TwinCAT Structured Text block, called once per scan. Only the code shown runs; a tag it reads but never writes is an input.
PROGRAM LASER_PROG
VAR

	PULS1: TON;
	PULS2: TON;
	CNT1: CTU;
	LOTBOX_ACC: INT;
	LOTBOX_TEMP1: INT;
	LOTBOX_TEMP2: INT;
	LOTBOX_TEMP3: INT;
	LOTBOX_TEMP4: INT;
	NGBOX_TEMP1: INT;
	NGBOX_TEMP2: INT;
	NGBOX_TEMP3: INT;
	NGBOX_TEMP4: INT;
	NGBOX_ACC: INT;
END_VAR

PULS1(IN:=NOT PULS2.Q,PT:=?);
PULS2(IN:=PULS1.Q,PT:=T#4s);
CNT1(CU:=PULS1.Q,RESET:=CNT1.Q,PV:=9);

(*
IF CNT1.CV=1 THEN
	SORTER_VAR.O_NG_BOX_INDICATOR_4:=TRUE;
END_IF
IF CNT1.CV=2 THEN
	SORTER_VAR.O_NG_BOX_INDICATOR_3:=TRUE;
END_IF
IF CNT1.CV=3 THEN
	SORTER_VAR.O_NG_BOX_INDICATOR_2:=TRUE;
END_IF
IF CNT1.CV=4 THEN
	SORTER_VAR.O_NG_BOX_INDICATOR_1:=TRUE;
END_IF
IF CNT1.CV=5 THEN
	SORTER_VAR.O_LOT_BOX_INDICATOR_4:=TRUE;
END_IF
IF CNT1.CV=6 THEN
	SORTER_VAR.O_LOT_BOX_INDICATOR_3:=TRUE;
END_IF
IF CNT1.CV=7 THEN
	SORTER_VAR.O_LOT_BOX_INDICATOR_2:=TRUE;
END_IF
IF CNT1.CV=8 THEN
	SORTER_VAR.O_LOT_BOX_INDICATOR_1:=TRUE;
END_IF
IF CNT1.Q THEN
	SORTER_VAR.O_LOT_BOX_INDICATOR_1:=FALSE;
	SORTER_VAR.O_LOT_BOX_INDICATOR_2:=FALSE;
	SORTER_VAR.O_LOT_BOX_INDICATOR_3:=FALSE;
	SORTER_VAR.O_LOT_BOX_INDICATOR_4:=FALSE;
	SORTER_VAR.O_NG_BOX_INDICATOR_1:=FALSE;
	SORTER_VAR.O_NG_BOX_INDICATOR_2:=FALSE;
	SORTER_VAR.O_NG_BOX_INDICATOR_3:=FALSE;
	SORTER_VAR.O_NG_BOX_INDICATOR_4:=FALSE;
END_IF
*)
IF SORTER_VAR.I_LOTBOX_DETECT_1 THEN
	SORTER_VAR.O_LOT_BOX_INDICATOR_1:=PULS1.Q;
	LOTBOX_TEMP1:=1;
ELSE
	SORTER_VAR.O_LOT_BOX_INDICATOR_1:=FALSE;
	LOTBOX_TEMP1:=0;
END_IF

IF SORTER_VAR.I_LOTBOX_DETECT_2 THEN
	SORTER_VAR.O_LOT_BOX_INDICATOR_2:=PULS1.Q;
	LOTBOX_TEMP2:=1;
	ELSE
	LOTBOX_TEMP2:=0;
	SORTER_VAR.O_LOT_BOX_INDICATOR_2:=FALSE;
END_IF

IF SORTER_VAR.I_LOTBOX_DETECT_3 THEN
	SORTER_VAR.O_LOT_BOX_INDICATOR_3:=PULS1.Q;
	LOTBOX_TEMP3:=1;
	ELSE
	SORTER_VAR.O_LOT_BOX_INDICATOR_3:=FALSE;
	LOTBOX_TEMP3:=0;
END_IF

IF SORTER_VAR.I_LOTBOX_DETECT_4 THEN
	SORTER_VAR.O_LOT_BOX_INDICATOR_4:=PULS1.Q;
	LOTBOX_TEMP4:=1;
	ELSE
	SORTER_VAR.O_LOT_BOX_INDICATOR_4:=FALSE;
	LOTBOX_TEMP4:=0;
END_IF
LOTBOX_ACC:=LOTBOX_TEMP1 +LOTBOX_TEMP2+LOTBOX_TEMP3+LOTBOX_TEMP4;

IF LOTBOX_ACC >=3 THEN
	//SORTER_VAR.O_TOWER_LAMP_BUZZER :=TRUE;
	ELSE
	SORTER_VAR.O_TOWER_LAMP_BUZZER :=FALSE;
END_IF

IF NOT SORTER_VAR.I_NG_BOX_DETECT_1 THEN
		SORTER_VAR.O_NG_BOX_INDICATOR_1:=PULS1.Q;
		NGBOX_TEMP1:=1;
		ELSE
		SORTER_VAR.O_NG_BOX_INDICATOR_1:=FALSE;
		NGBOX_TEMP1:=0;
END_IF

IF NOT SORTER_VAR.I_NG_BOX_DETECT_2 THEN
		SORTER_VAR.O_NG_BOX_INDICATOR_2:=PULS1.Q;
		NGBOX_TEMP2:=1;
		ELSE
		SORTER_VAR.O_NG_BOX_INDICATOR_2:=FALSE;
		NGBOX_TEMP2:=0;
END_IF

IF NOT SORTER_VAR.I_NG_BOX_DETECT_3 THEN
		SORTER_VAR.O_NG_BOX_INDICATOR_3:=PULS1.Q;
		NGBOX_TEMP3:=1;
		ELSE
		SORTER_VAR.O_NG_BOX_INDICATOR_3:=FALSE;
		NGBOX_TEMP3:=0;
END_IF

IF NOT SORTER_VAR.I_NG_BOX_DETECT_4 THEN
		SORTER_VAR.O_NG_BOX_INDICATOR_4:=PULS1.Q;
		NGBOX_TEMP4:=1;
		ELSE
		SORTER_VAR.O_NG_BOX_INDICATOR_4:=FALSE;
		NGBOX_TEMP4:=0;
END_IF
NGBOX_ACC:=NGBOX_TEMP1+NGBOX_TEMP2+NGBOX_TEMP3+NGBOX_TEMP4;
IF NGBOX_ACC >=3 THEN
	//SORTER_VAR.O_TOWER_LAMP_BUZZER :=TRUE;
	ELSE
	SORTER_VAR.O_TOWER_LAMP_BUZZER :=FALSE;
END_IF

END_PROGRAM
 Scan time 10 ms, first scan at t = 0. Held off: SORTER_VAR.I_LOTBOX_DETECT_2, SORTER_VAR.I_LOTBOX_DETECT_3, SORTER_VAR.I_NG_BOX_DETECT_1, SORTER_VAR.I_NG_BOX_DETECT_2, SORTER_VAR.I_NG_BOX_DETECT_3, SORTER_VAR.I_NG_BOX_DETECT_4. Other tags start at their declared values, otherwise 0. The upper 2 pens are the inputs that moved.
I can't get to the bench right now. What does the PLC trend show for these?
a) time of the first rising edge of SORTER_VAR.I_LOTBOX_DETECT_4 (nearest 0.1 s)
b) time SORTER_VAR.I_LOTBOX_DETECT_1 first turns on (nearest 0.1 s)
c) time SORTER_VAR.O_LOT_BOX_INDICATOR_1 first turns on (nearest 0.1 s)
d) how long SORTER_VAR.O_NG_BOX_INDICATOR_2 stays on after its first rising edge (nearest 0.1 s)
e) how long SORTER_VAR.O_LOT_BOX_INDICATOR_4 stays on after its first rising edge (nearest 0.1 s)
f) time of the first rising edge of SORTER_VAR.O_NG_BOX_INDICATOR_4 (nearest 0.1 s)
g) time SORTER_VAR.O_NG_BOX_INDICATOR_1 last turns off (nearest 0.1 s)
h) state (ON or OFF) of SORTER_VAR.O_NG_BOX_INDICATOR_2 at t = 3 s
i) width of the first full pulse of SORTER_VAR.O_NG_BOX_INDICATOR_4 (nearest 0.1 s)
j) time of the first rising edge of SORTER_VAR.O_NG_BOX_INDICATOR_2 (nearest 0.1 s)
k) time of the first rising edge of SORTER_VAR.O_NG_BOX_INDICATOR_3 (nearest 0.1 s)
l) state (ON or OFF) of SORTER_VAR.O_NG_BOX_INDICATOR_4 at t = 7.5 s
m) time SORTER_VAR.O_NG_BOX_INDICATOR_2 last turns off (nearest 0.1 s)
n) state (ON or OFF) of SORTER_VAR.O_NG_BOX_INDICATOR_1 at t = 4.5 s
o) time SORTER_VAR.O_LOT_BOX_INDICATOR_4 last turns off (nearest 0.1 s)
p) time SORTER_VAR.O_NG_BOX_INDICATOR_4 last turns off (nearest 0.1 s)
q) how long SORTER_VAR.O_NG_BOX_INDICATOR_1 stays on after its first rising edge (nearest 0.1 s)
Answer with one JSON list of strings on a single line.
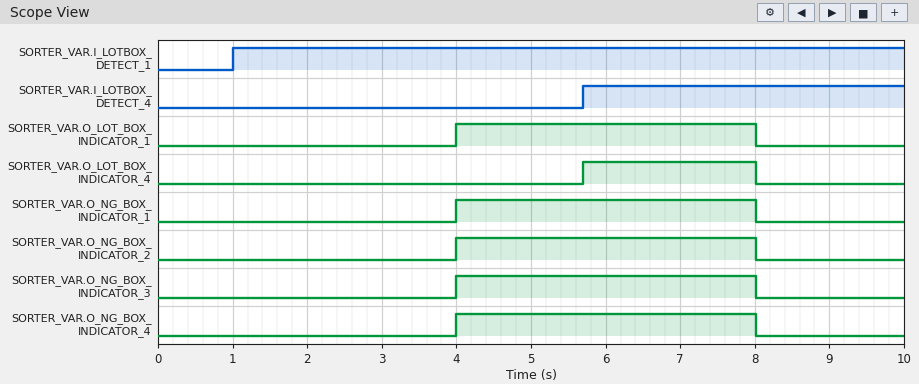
["5.7 s", "1.0 s", "4.0 s", "4.0 s", "2.3 s", "4.0 s", "8.0 s", "OFF", "4.0 s", "4.0 s", "4.0 s", "ON", "8.0 s", "ON", "8.0 s", "8.0 s", "4.0 s"]
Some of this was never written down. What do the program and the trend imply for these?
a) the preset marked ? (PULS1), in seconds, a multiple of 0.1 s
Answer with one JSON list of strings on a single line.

["4.0 s"]
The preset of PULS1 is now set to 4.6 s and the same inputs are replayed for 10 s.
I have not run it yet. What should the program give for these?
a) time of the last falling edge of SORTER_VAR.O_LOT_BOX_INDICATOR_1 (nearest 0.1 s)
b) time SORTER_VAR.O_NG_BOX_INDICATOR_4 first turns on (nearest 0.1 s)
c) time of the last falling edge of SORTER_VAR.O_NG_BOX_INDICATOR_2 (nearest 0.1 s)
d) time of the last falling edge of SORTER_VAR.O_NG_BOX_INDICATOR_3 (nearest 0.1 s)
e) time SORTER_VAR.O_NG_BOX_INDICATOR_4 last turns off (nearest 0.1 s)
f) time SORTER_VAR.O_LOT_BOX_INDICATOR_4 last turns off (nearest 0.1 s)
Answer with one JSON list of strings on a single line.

["8.6 s", "4.6 s", "8.6 s", "8.6 s", "8.6 s", "8.6 s"]
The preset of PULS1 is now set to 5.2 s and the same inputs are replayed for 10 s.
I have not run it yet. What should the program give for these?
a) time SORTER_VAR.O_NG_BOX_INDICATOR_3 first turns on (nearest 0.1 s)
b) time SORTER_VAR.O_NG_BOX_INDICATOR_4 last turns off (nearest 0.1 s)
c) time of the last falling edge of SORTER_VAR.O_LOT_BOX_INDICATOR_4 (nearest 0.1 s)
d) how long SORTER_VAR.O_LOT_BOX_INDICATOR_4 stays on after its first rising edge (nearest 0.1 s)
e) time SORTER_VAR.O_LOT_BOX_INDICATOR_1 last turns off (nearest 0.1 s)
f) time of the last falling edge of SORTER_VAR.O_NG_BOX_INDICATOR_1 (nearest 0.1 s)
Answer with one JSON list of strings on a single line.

["5.2 s", "9.2 s", "9.2 s", "3.5 s", "9.2 s", "9.2 s"]
